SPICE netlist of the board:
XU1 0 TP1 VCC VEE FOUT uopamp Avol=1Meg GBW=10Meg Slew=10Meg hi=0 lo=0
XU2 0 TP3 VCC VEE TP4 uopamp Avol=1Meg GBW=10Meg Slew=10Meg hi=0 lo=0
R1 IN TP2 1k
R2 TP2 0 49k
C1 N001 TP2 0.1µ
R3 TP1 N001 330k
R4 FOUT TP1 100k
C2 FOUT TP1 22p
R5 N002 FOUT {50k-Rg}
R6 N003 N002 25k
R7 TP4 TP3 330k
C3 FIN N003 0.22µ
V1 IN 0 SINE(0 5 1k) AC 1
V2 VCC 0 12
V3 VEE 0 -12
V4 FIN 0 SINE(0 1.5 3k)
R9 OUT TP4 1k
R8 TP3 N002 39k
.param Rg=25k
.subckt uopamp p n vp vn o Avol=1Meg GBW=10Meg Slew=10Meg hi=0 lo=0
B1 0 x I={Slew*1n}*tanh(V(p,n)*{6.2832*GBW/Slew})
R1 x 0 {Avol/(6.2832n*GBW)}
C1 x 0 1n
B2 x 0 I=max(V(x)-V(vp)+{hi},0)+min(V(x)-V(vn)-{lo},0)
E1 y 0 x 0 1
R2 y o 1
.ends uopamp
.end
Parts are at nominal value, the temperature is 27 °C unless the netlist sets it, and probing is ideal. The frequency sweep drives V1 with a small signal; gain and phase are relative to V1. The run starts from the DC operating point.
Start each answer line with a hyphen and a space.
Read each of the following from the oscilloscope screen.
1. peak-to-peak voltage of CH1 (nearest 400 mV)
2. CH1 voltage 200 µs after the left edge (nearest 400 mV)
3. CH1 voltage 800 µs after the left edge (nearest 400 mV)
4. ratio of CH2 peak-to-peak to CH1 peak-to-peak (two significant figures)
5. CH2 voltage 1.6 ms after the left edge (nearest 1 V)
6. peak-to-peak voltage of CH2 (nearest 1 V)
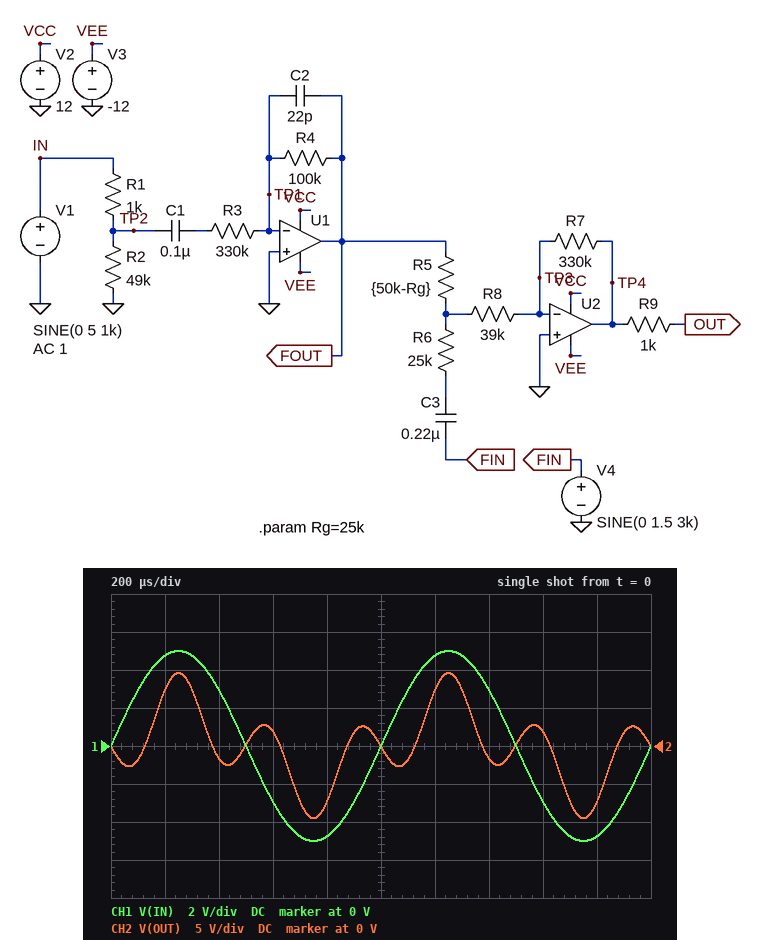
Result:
- 10.0 V
- 4.8 V
- -4.8 V
- 1.9
- 2 V
- 19 V
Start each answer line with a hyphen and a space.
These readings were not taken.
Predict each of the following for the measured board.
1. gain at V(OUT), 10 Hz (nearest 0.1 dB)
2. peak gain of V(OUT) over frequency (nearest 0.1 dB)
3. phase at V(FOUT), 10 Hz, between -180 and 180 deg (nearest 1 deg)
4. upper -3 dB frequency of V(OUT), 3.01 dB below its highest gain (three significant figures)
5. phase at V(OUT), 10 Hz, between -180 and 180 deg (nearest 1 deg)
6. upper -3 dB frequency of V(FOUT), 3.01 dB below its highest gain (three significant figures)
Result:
- 2.1 dB
- 2.1 dB
- -154 deg
- 23.2 kHz
- 16 deg
- 72.2 kHz
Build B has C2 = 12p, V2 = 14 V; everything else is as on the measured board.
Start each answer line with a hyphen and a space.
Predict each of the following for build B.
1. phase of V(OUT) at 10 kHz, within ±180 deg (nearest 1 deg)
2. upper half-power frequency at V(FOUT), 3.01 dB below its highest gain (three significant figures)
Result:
- -5 deg
- 132 kHz
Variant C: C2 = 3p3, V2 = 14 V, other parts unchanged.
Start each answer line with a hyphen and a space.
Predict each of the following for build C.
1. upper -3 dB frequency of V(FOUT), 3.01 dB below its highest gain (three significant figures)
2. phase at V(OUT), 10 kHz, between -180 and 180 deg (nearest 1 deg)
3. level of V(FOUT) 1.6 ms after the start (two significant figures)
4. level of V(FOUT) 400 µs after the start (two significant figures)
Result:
- 474 kHz
- -2 deg
- 880 mV
- -860 mV
